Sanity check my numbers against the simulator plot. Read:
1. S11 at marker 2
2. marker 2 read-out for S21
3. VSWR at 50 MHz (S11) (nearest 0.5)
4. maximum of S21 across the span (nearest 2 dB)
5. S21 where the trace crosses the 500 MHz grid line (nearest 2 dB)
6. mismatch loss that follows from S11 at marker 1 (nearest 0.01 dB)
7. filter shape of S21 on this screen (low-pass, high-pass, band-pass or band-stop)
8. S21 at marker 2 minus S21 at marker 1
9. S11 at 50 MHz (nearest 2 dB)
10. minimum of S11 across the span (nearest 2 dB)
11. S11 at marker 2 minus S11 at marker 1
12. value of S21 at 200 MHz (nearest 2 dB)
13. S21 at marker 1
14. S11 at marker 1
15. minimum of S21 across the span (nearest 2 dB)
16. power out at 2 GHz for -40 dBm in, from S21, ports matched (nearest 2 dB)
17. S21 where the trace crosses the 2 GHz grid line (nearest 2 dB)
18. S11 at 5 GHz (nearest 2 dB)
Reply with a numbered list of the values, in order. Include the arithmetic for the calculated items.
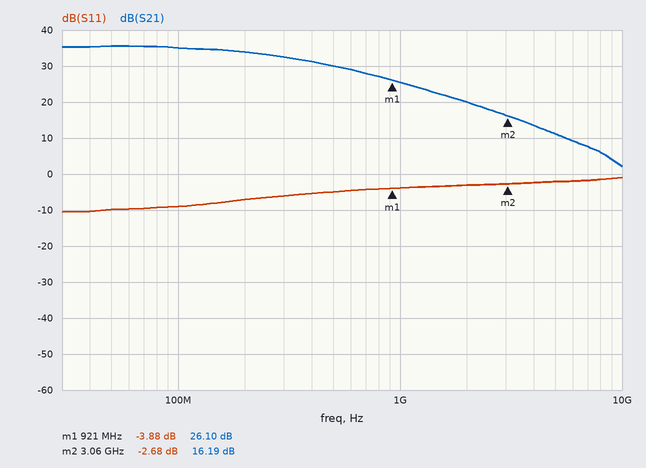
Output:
1. -2.68 dB
2. 16.19 dB
3. |Γ| = 10^(-10/20) = 0.3162; VSWR = (1 + 0.3162)/(1 − 0.3162) ≈ 1.92, so 2.0 to the nearest 0.5
4. 36 dB
5. 30 dB
6. −10 log10(1 − 10^(-3.88/10)) ≈ 2.29 dB
7. low-pass
8. 16.19 − (26.1) = -9.91 dB
9. -10 dB
10. -10 dB
11. -2.68 − (-3.88) = 1.20 dB
12. 34 dB
13. 26.10 dB
14. -3.88 dB
15. 2 dB
16. -40 dBm + (20 dB) = -20 dBm
17. 20 dB
18. -2 dB
